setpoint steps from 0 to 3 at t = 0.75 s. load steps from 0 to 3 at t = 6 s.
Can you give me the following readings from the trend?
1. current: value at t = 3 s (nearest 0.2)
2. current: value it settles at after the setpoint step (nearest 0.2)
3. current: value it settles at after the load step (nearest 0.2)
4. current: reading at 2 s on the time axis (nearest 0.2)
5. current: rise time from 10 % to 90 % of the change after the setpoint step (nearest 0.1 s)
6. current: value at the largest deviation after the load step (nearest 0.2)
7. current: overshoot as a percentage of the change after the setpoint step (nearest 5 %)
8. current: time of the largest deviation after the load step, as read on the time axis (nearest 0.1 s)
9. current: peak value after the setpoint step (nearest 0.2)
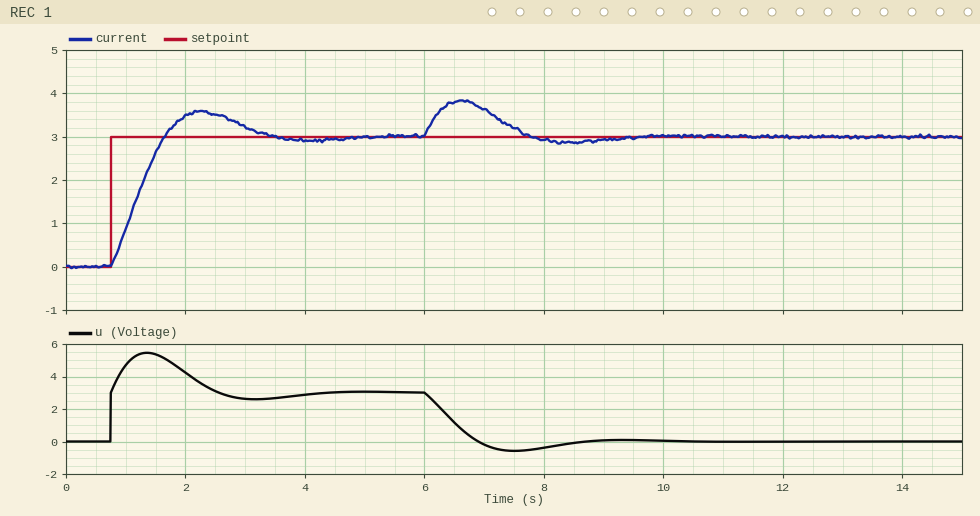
3.2
3.0
3.0
3.4
0.7 s
3.8
20 %
6.6 s
3.6
